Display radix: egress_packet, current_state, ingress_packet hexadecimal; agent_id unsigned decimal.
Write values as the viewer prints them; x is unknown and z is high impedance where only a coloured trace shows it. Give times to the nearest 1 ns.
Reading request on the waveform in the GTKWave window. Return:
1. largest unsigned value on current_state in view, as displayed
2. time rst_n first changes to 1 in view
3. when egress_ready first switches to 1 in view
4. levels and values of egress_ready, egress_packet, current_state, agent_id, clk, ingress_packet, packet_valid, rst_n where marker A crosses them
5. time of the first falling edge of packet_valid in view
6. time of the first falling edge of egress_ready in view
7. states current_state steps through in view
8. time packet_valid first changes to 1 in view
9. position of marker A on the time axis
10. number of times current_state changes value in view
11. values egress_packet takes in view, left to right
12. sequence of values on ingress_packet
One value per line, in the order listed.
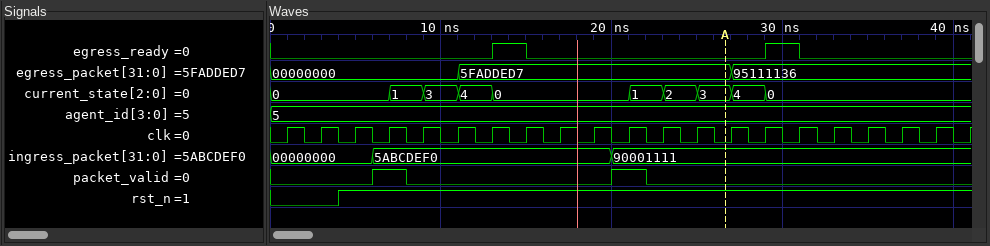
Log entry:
4
4 ns
13 ns
egress_ready=0, egress_packet=5FADDED7, current_state=3, agent_id=5, clk=0, ingress_packet=90001111, packet_valid=0, rst_n=1
8 ns
15 ns
0, 1, 3, 4, 0, 1, 2, 3, 4, 0
6 ns
27 ns
9
00000000, 5FADDED7, 95111136
00000000, 5ABCDEF0, 90001111
